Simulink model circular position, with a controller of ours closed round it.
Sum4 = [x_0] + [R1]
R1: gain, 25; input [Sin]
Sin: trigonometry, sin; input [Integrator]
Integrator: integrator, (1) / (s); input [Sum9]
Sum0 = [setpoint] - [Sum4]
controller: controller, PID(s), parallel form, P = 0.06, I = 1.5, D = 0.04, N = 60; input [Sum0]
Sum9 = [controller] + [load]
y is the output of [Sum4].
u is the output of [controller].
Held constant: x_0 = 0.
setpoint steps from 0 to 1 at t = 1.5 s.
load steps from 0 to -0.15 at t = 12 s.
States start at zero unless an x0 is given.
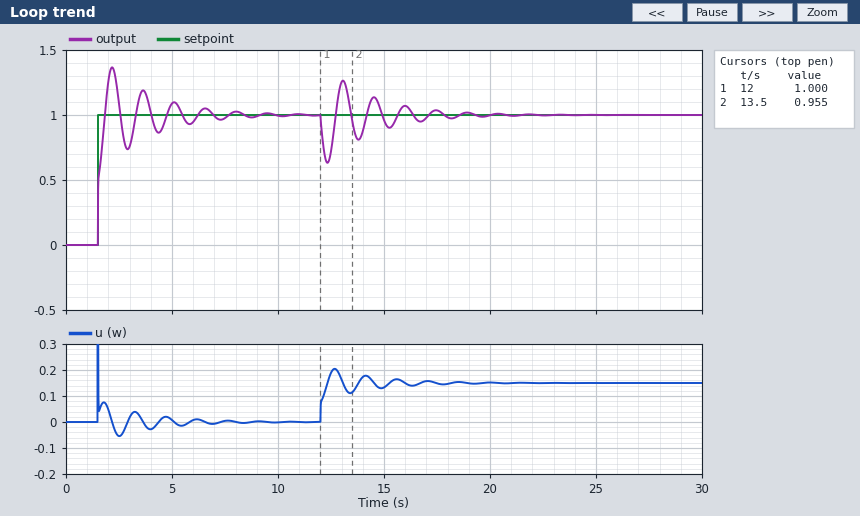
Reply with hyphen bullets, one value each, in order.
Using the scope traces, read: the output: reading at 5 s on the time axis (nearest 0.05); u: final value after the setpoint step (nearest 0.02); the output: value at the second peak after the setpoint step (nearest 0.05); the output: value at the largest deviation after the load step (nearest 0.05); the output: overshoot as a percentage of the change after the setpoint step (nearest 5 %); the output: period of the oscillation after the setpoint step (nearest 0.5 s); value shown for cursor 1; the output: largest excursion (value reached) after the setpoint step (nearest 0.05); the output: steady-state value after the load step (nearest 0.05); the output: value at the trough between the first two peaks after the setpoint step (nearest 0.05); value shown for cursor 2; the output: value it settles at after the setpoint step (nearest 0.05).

- 1.10
- 0.00
- 1.20
- 0.65
- 35 %
- 1.5 s
- 1.000
- 1.35
- 1.00
- 0.75
- 0.955
- 1.00
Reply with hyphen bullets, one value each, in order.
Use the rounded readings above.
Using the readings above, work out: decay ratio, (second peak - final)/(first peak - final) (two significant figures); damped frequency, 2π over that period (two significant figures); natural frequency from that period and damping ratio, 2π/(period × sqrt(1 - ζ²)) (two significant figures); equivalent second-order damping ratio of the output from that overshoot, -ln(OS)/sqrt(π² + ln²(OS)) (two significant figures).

- 0.57
- 4.2 rad/s
- 4.4 rad/s
- 0.32
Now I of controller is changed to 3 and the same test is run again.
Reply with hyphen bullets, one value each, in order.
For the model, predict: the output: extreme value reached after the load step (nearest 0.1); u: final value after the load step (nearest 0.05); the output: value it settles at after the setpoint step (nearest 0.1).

- 0.7
- 0.15
- 1.0
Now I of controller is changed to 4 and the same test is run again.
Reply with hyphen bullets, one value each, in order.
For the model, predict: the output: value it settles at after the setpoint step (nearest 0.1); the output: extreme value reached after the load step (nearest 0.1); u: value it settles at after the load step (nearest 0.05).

- 1.0
- 0.8
- 0.15
